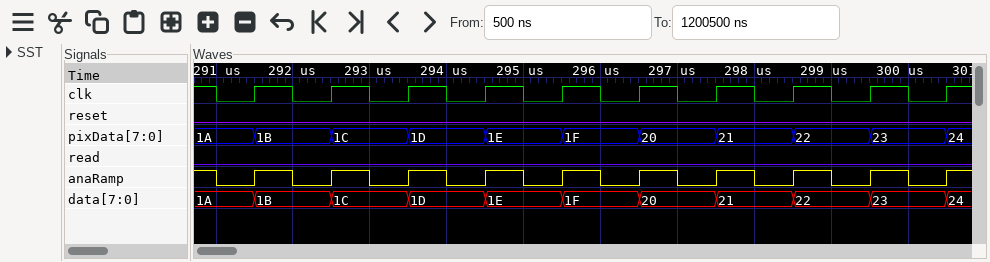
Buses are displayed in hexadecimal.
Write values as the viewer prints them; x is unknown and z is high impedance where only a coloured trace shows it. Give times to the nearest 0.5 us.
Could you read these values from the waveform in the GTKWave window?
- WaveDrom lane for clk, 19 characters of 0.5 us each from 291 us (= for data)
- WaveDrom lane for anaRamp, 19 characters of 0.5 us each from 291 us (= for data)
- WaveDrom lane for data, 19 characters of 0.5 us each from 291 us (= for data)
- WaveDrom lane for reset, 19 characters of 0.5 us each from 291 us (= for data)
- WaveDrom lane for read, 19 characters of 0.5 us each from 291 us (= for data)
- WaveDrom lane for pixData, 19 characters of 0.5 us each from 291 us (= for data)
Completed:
{name: 'clk', wave: '0101010101010101010'}
{name: 'anaRamp', wave: '0101010101010101010'}
{name: 'data', wave: '==.=.=.=.=.=.=.=.=.', data: '1A 1B 1C 1D 1E 1F 20 21 22 23'}
{name: 'reset', wave: '0..................'}
{name: 'read', wave: '0..................'}
{name: 'pixData', wave: '==.=.=.=.=.=.=.=.=.', data: '1A 1B 1C 1D 1E 1F 20 21 22 23'}
